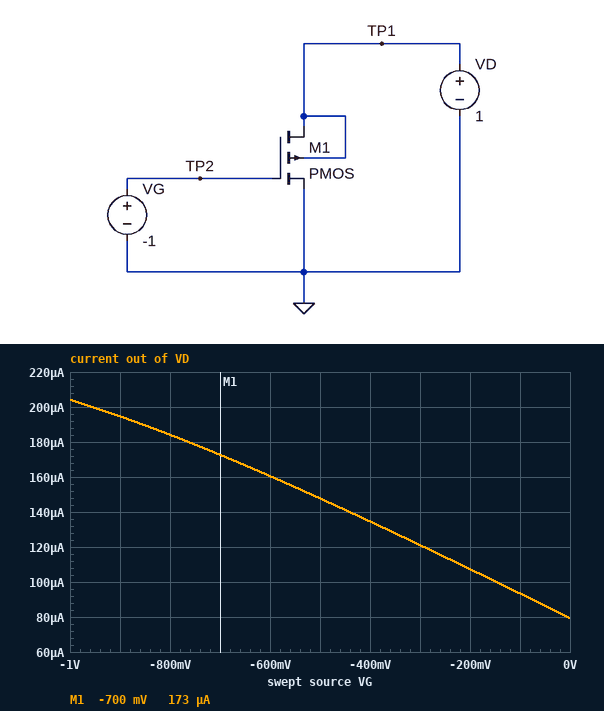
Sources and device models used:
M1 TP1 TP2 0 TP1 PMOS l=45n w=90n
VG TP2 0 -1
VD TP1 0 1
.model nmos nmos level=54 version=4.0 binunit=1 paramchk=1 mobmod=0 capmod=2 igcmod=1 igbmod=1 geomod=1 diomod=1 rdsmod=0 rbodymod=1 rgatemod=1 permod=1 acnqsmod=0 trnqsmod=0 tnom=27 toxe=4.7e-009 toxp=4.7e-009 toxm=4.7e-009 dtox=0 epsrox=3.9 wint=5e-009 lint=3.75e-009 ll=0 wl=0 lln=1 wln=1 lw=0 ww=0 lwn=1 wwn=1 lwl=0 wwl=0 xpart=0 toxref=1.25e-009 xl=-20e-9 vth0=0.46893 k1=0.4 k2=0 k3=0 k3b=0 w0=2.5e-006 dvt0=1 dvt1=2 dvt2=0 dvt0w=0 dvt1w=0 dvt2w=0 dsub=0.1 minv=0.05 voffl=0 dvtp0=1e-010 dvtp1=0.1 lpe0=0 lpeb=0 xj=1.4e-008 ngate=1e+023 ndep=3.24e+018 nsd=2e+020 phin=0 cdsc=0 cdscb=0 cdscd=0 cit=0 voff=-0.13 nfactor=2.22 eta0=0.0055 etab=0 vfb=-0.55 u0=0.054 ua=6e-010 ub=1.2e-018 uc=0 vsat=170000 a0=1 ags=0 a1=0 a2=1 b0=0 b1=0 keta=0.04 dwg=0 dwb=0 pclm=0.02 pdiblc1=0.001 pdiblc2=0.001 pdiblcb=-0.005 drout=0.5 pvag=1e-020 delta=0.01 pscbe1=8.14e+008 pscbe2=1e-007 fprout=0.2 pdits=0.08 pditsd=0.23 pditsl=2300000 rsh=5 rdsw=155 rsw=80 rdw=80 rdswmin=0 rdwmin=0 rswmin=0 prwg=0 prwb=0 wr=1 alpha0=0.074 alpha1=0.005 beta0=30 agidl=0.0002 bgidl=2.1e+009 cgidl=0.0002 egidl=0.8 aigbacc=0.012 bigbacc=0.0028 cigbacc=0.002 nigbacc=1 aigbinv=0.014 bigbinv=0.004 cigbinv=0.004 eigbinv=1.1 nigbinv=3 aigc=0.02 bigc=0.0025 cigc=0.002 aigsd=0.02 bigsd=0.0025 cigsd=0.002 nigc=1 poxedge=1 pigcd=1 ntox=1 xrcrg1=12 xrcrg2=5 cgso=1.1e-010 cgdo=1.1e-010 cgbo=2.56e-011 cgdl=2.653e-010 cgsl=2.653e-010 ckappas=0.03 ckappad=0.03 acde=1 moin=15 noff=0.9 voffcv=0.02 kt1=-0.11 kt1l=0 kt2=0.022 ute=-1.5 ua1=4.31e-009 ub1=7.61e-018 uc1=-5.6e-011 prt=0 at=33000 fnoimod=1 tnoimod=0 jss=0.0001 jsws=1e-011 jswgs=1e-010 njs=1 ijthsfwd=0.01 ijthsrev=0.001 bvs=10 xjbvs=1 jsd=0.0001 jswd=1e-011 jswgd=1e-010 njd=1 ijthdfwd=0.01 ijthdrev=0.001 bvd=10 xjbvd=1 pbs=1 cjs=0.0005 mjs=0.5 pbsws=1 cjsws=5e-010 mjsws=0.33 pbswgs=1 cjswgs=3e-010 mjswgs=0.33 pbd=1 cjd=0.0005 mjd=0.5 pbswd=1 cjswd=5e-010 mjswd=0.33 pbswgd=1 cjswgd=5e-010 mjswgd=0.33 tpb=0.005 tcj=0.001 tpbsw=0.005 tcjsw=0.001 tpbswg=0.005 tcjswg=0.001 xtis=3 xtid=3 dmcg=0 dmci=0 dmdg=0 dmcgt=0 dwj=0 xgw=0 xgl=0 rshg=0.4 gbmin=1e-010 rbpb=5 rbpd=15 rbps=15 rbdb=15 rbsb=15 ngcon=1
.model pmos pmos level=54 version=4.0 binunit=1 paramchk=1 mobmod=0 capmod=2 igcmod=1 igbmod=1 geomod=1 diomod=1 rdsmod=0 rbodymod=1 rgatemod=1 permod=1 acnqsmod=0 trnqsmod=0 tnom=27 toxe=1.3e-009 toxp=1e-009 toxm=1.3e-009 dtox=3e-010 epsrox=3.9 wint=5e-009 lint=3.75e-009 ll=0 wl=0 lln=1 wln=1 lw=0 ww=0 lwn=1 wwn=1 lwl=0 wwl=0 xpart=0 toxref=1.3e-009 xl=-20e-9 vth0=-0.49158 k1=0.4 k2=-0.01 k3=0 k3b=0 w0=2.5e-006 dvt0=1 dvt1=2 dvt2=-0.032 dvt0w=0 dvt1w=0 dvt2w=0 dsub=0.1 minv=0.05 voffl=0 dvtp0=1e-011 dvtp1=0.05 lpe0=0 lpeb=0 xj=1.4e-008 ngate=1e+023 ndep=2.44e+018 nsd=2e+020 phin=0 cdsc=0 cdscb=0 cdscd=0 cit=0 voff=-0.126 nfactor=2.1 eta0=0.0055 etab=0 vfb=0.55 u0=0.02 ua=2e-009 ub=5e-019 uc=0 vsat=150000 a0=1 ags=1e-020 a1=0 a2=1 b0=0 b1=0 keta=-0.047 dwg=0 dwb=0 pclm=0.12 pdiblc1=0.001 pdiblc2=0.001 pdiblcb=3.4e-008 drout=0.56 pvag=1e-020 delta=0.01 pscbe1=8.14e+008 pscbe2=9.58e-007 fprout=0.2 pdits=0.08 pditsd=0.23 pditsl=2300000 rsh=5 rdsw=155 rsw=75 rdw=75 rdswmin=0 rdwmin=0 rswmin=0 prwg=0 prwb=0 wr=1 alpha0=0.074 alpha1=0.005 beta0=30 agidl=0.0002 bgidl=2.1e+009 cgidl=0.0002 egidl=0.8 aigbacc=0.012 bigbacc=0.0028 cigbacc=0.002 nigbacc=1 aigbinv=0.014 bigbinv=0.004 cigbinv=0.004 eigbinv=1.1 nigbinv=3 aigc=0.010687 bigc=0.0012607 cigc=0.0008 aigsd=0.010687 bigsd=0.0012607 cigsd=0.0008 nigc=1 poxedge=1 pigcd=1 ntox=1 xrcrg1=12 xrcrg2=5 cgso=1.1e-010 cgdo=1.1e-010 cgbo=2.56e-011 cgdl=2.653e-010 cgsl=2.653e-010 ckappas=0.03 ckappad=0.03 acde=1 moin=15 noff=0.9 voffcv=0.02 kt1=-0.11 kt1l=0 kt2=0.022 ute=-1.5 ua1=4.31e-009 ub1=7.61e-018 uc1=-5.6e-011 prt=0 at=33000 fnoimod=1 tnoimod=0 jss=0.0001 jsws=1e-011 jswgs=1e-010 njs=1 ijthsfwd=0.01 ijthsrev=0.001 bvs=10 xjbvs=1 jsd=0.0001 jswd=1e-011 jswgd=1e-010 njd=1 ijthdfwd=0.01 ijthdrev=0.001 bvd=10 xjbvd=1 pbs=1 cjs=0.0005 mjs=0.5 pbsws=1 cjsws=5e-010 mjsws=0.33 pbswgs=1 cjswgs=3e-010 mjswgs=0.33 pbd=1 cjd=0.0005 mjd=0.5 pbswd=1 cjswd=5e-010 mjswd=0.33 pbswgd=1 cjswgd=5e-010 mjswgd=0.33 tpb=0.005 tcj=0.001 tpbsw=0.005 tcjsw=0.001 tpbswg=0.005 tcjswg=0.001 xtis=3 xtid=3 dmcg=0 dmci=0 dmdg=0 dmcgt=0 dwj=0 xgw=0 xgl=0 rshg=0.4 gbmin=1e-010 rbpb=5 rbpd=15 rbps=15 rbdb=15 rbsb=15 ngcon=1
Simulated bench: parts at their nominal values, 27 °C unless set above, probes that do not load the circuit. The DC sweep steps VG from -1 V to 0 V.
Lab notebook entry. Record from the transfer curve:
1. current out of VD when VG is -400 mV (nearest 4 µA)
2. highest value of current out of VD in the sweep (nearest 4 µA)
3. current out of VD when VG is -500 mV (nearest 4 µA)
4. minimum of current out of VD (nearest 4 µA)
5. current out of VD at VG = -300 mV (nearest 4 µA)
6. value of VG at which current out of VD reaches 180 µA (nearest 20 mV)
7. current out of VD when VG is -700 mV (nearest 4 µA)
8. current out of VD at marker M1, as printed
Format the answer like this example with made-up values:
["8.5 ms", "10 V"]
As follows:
["136 µA", "204 µA", "148 µA", "80 µA", "120 µA", "-760 mV", "172 µA", "173 µA"]
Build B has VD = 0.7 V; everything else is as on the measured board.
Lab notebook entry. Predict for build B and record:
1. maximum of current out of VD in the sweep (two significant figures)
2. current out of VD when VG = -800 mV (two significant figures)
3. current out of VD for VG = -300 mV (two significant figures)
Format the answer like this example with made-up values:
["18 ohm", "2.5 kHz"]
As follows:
["140 µA", "130 µA", "69 µA"]
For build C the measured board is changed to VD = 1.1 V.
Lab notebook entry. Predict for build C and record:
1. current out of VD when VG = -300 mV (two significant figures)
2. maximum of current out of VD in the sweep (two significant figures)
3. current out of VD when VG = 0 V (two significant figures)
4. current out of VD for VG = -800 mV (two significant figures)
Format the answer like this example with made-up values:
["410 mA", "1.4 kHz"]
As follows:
["140 µA", "220 µA", "97 µA", "200 µA"]
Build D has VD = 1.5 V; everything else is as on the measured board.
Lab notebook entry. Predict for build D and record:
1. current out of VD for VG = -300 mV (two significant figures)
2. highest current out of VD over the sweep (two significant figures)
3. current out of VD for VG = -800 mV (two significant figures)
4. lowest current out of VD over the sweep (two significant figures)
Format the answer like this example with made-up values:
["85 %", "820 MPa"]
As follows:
["210 µA", "310 µA", "280 µA", "170 µA"]
